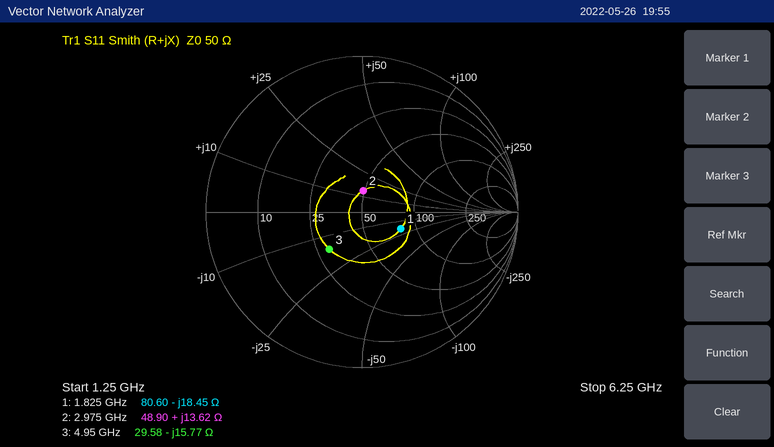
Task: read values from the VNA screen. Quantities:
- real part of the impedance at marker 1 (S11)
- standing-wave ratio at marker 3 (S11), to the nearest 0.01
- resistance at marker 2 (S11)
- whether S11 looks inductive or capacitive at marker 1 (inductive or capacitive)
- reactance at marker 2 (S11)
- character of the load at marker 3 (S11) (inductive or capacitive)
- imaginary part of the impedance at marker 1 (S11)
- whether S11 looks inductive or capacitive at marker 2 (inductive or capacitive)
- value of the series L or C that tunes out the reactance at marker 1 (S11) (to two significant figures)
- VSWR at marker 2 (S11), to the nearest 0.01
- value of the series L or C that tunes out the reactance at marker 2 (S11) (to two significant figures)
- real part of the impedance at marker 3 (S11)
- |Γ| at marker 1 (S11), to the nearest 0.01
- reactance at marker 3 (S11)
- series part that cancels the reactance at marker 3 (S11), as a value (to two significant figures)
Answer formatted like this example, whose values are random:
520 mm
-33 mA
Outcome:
80.60 Ω
1.93
48.90 Ω
capacitive
+13.62 Ω
capacitive
-18.45 Ω
inductive
1.6 nH
1.32
3.9 pF
29.58 Ω
0.27
-15.77 Ω
510 pH
